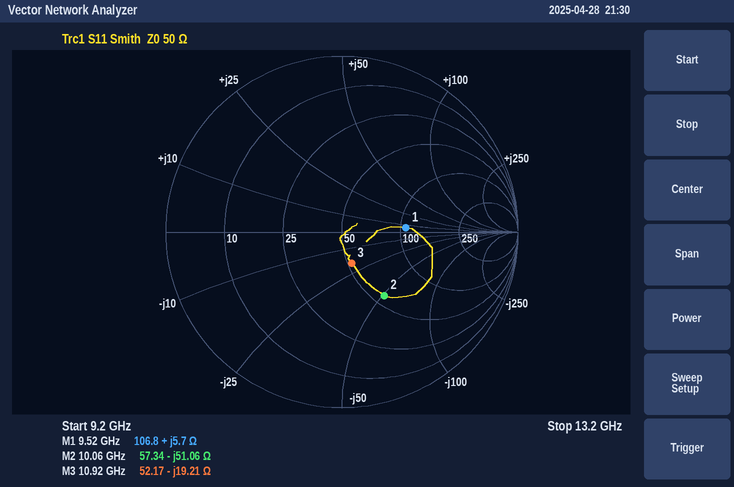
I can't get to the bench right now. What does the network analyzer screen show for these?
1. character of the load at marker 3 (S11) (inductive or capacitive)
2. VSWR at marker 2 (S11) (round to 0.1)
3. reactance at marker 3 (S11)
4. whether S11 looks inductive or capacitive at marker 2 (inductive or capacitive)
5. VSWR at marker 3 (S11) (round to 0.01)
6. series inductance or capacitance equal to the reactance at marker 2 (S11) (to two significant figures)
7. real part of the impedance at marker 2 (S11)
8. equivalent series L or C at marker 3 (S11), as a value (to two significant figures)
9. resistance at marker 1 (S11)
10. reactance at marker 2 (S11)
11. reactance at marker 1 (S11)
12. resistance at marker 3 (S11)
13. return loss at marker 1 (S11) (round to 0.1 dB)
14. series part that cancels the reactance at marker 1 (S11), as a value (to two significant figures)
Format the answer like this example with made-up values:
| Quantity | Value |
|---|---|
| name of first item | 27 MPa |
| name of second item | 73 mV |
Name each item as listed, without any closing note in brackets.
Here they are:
| Quantity | Value |
|---|---|
| character of the load at marker 3 (S11) | capacitive |
| VSWR at marker 2 (S11) | 2.5 |
| reactance at marker 3 | -19.21 Ω |
| whether S11 looks inductive or capacitive at marker 2 | capacitive |
| VSWR at marker 3 (S11) | 1.46 |
| series inductance or capacitance equal to the reactance at marker 2 (S11) | 310 fF |
| real part of the impedance at marker 2 | 57.34 Ω |
| equivalent series L or C at marker 3 (S11), as a value | 760 fF |
| resistance at marker 1 | 106.8 Ω |
| reactance at marker 2 | -51.06 Ω |
| reactance at marker 1 | +5.7 Ω |
| resistance at marker 3 | 52.17 Ω |
| return loss at marker 1 (S11) | 8.8 dB |
| series part that cancels the reactance at marker 1 (S11), as a value | 2.9 pF |
